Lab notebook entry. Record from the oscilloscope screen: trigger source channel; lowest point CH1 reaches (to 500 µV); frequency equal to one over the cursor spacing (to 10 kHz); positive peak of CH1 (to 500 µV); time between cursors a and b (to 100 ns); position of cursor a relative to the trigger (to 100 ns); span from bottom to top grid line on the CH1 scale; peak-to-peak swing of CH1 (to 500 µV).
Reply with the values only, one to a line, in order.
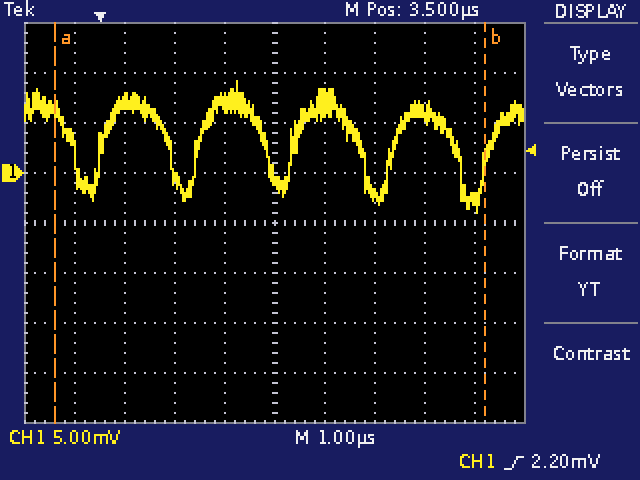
CH1
-4.0 mV
120 kHz
9.0 mV
8.6 µs
-900 ns
40 mV
13.0 mV
